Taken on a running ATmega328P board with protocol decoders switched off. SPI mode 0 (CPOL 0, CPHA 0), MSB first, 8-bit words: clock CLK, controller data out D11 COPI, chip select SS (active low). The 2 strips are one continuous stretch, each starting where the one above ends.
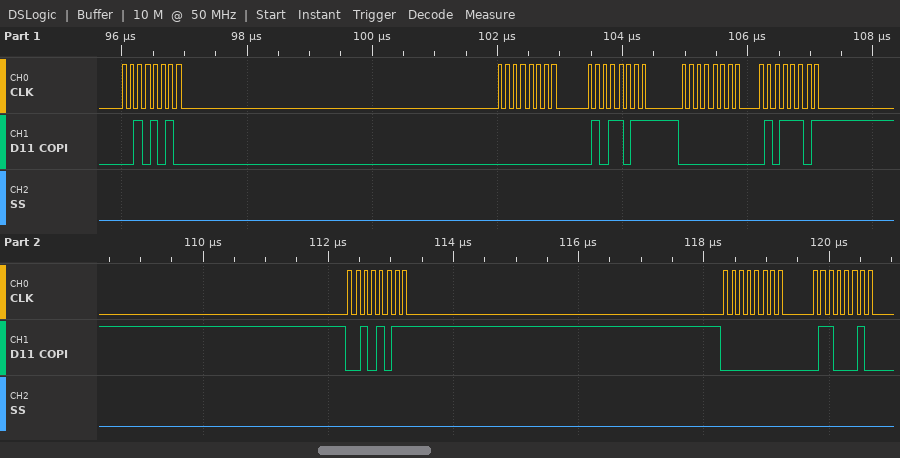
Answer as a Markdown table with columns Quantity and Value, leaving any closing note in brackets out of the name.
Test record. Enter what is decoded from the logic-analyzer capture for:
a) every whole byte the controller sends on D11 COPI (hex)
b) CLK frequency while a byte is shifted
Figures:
| Quantity | Value |
|---|---|
| every whole byte the controller sends on D11 COPI | 2A 00 5B 00 5D 2B 00 62 |
| CLK frequency while a byte is shifted | 8 MHz |
